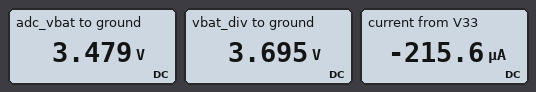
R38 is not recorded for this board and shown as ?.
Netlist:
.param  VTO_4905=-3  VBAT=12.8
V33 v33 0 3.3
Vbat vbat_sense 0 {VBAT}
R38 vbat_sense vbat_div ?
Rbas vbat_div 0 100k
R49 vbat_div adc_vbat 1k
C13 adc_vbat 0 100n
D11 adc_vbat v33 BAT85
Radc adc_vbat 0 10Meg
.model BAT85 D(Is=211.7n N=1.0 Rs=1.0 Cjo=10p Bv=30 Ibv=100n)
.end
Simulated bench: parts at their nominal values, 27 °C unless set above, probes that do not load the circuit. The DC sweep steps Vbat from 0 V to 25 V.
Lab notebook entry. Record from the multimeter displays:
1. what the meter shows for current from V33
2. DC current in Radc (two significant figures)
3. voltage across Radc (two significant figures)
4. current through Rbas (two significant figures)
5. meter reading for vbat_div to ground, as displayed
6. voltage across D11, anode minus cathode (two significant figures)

-215.6 µA
350 nA
3.5 V
37 µA
3.695 V
180 mV
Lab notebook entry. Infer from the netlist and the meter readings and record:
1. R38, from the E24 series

36 kΩ
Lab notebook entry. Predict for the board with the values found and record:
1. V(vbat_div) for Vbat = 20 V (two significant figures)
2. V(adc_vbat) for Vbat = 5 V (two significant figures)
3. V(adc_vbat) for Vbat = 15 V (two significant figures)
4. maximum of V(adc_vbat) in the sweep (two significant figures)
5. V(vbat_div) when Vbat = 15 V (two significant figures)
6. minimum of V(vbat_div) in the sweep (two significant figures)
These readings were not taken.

3.9 V
3.4 V
3.5 V
3.5 V
3.8 V
5.6 mV
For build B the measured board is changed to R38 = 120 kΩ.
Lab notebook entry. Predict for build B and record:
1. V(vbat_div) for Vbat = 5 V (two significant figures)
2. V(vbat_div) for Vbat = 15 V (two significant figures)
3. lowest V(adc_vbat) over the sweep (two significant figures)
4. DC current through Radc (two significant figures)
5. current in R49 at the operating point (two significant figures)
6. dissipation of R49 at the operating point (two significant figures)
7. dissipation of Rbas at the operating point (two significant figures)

2.3 V
3.5 V
12 mV
340 nA
43 µA
1.8 µW
120 µW
